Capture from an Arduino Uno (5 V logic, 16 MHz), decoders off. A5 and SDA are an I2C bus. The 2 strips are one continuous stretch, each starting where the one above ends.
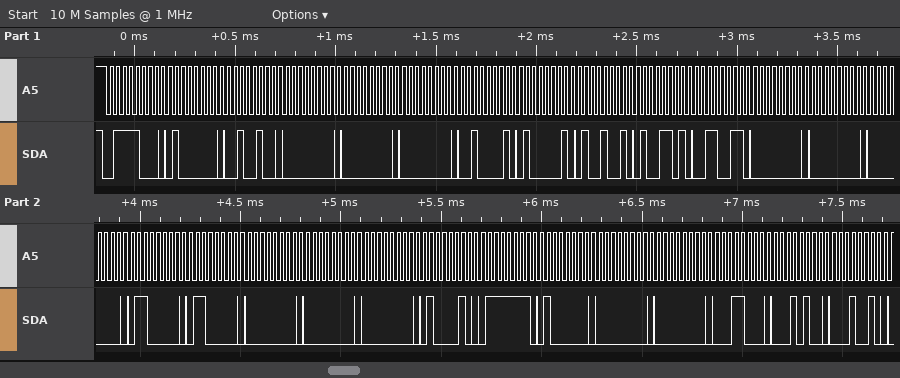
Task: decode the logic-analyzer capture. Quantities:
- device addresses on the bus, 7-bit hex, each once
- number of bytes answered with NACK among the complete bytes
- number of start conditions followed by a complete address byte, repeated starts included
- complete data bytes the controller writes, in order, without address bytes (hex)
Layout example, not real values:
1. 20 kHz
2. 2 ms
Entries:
1. 0x3C
2. 0
3. 1
4. 40 24 00 00 00 21 41 49 4D 33 00 00 00 60 60 00 00 00 42 7F 40 00 00 18 14 12
